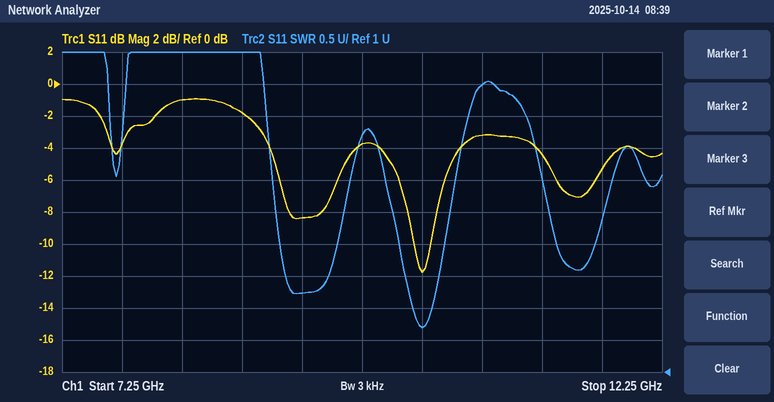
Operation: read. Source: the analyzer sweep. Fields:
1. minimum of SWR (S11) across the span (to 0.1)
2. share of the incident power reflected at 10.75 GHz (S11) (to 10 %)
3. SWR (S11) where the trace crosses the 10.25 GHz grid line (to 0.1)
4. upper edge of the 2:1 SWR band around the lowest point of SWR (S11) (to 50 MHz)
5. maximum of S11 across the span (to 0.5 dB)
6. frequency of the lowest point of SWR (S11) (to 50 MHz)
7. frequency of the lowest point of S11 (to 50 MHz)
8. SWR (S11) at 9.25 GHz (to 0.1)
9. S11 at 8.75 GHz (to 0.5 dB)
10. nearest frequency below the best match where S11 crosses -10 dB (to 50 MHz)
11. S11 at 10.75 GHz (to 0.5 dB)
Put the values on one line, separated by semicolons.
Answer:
1.7; 50 %; 1.7; 10.35 GHz; -1.0 dB; 10.25 GHz; 10.25 GHz; 2.2; -2.0 dB; 10.20 GHz; -3.0 dB
